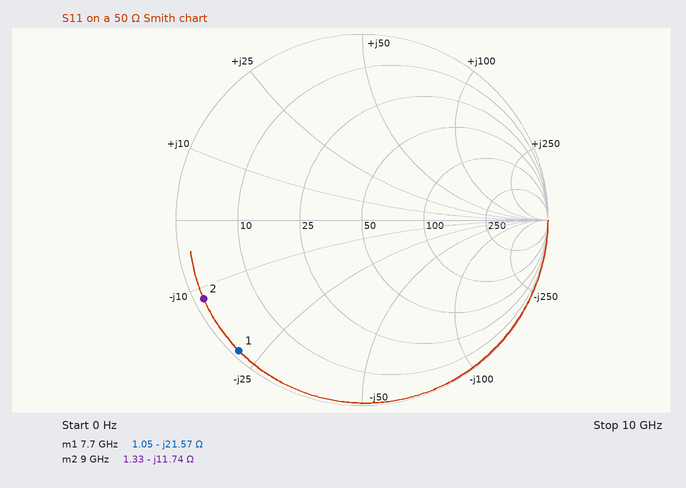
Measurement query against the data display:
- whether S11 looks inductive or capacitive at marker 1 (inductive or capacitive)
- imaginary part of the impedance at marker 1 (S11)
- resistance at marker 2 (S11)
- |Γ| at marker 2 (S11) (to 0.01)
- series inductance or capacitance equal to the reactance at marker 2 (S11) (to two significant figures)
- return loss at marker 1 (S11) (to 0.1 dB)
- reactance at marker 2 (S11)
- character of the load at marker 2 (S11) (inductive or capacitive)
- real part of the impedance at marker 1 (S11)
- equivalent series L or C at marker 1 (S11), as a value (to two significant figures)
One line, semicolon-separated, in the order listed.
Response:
capacitive; -21.57 Ω; 1.33 Ω; 0.95; 1.5 pF; 0.3 dB; -11.74 Ω; capacitive; 1.05 Ω; 960 fF
